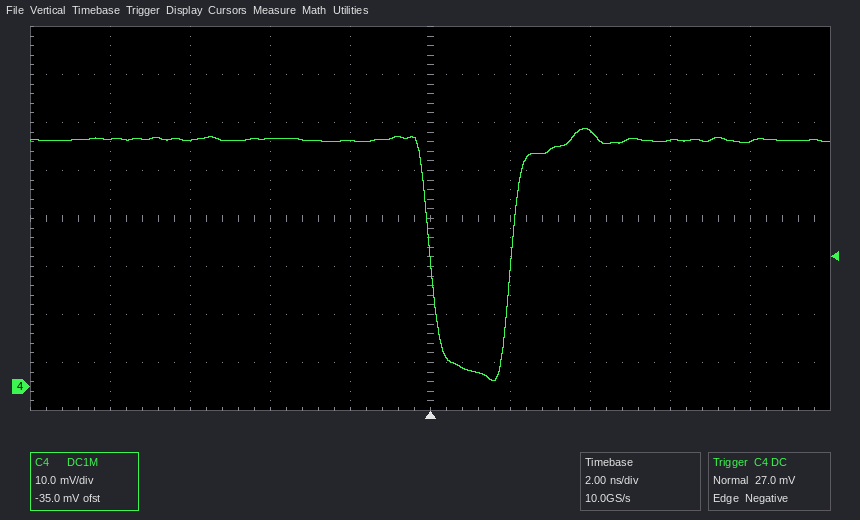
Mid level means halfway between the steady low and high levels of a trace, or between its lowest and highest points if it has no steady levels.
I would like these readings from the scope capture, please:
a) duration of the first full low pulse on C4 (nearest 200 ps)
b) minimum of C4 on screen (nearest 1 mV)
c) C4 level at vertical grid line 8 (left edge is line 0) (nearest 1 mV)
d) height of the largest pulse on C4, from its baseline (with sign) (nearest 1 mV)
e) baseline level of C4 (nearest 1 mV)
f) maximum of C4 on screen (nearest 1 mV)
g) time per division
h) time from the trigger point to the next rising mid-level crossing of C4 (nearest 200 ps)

2.0 ns
1 mV
51 mV
-50 mV
51 mV
54 mV
2 ns
2.0 ns
